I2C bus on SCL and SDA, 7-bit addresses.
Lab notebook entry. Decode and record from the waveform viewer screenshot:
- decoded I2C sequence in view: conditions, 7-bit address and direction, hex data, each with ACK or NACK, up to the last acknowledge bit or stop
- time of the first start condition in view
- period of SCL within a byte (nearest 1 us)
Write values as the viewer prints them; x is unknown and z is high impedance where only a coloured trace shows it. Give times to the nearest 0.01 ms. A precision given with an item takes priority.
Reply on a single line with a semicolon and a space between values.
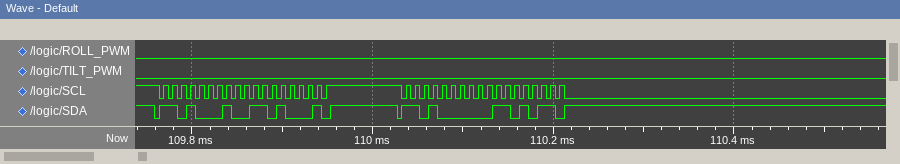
start, address 68 read ACK, 68 NACK, stop, start, address 68 write ACK, 6B ACK; 109.76 ms; 10 us
